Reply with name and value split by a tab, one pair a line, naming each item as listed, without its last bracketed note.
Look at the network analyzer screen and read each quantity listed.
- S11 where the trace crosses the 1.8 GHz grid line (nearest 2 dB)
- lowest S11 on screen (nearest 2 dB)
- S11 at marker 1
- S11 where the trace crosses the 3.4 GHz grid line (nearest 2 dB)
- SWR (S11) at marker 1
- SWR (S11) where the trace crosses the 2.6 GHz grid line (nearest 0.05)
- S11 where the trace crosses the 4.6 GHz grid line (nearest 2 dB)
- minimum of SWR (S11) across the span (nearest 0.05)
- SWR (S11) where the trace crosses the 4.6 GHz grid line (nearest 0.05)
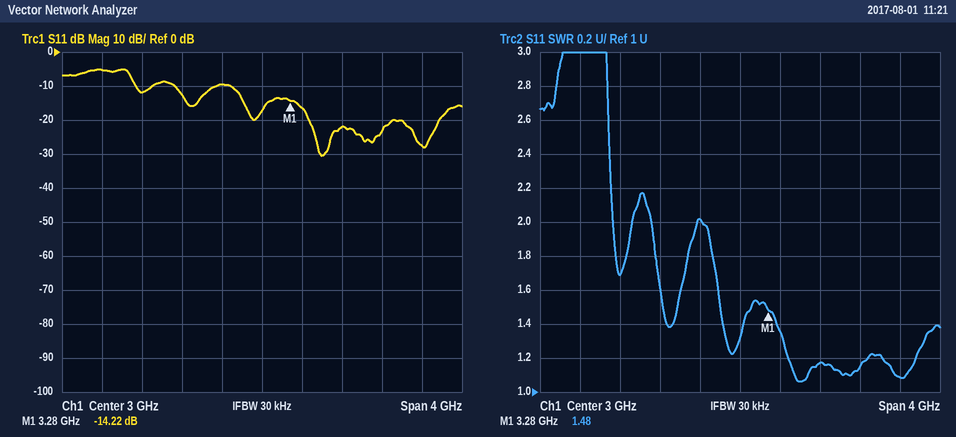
S11 where the trace crosses the 1.8 GHz grid line	-12 dB
lowest S11 on screen	-30 dB
S11 at marker 1	-14.22 dB
S11 where the trace crosses the 3.4 GHz grid line	-16 dB
SWR (S11) at marker 1	1.48
SWR (S11) where the trace crosses the 2.6 GHz grid line	2.00
S11 where the trace crosses the 4.6 GHz grid line	-28 dB
minimum of SWR (S11) across the span	1.05
SWR (S11) where the trace crosses the 4.6 GHz grid line	1.10
